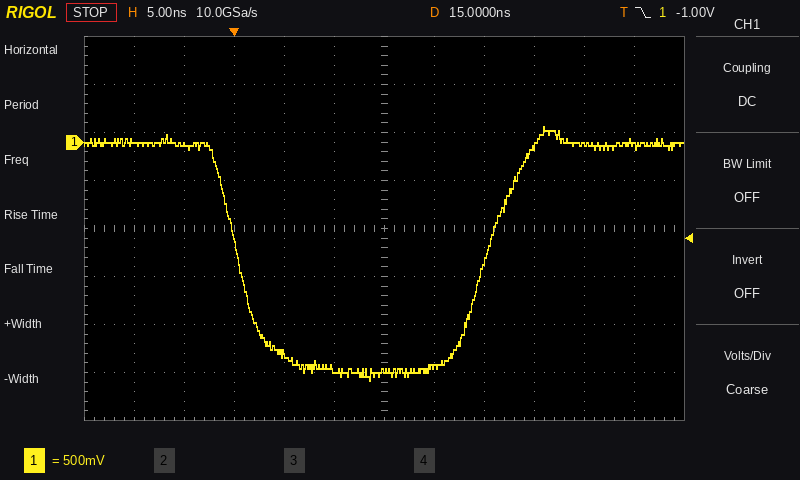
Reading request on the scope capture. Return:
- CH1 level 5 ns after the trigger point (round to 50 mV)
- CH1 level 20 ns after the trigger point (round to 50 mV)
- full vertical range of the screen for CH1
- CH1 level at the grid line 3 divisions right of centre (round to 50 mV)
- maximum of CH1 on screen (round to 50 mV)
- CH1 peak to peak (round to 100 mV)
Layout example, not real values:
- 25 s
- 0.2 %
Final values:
- -2.20 V
- -2.35 V
- 4 V
- -50 mV
- 150 mV
- 2.60 V
